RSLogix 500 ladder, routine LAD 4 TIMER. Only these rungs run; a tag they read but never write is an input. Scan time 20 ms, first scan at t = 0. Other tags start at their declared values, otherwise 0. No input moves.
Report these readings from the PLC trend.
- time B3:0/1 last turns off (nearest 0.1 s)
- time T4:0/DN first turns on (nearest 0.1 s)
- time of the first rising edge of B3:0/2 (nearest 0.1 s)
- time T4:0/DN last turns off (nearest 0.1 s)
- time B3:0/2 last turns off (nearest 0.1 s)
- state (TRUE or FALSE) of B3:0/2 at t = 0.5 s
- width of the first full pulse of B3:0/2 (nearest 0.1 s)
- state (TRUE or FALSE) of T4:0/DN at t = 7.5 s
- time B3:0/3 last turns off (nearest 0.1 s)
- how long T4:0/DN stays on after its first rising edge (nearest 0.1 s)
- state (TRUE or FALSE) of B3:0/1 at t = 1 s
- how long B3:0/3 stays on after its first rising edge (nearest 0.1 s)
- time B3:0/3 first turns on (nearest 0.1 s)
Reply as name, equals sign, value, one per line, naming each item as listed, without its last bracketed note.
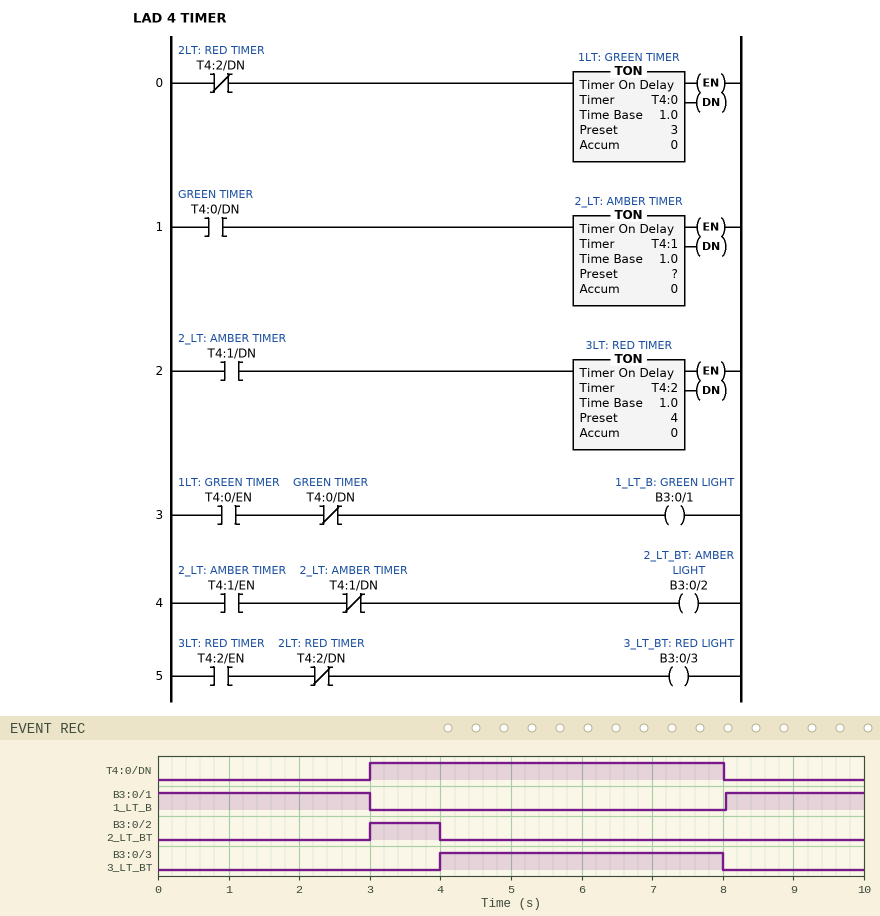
time B3:0/1 last turns off = 3.0 s
time T4:0/DN first turns on = 3.0 s
time of the first rising edge of B3:0/2 = 3.0 s
time T4:0/DN last turns off = 8.0 s
time B3:0/2 last turns off = 4.0 s
state (TRUE or FALSE) of B3:0/2 at t = 0.5 s = FALSE
width of the first full pulse of B3:0/2 = 1.0 s
state (TRUE or FALSE) of T4:0/DN at t = 7.5 s = TRUE
time B3:0/3 last turns off = 8.0 s
how long T4:0/DN stays on after its first rising edge = 5.0 s
state (TRUE or FALSE) of B3:0/1 at t = 1 s = TRUE
how long B3:0/3 stays on after its first rising edge = 4.0 s
time B3:0/3 first turns on = 4.0 s
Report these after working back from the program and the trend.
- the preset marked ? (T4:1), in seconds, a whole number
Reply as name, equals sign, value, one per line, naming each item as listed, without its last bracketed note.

the preset marked ? (T4:1), in seconds, a whole number = 1 s
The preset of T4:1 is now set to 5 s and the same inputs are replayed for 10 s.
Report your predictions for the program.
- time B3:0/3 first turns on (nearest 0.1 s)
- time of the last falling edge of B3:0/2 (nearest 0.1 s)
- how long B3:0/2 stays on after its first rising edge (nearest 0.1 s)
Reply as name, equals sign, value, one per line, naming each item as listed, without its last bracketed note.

time B3:0/3 first turns on = 8.0 s
time of the last falling edge of B3:0/2 = 8.0 s
how long B3:0/2 stays on after its first rising edge = 5.0 s
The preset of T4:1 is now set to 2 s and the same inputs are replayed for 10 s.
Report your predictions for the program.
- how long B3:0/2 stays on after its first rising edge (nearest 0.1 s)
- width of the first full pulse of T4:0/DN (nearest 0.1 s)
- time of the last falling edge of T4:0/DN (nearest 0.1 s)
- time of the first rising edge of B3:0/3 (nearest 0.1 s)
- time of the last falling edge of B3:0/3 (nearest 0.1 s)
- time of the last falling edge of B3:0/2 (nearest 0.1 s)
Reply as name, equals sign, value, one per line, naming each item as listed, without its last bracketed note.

how long B3:0/2 stays on after its first rising edge = 2.0 s
width of the first full pulse of T4:0/DN = 6.0 s
time of the last falling edge of T4:0/DN = 9.0 s
time of the first rising edge of B3:0/3 = 5.0 s
time of the last falling edge of B3:0/3 = 9.0 s
time of the last falling edge of B3:0/2 = 5.0 s
